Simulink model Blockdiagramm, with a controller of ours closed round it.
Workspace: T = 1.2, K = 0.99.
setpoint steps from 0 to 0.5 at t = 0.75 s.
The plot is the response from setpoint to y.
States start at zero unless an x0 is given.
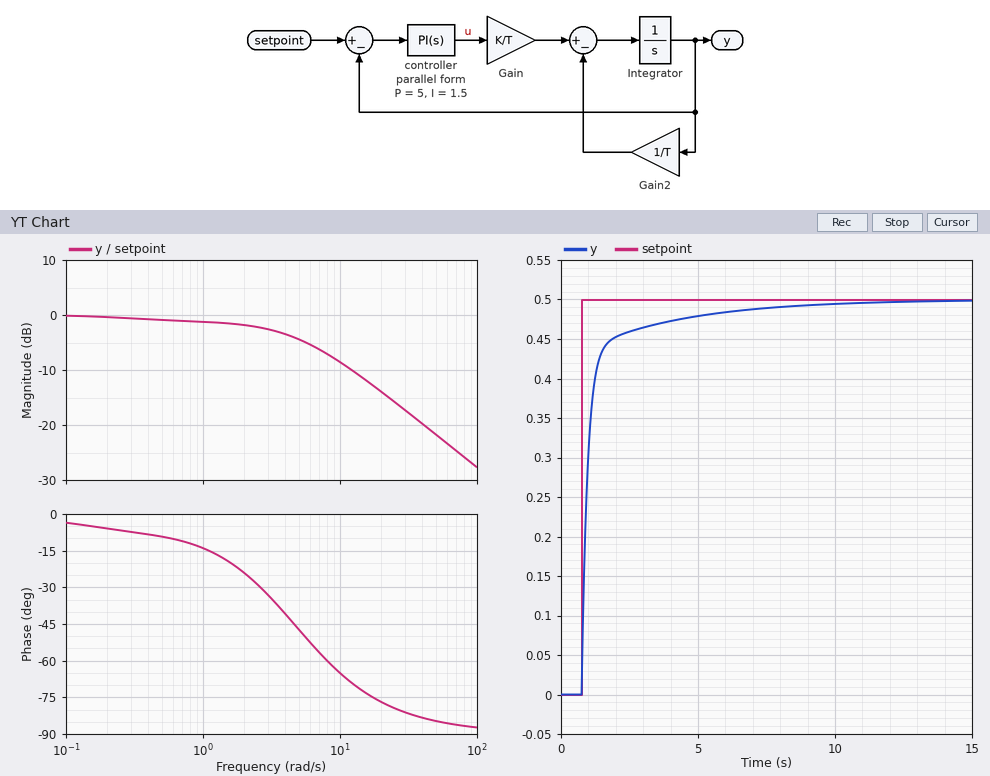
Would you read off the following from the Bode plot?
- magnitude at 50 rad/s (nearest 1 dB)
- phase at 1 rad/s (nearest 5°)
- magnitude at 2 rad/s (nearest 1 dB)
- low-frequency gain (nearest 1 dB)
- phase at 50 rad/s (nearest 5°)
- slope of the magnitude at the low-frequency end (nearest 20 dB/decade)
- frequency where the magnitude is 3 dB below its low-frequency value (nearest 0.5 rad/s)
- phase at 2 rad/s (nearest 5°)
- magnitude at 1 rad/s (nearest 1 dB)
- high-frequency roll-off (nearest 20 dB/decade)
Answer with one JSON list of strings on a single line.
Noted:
["-22 dB", "-15°", "-2 dB", "0 dB", "-85°", "0 dB/decade", "3.5 rad/s", "-25°", "-1 dB", "-20 dB/decade"]
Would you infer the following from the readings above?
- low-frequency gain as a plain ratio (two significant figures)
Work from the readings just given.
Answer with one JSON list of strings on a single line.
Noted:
["1.0"]
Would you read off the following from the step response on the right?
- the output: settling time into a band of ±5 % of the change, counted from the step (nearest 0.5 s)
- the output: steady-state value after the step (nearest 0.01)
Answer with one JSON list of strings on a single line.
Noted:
["3.5 s", "0.50"]
